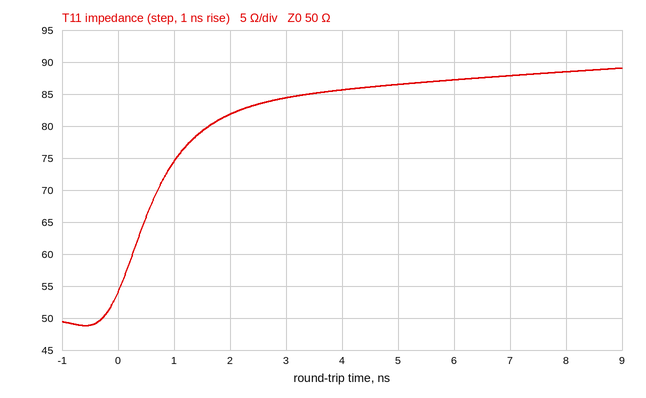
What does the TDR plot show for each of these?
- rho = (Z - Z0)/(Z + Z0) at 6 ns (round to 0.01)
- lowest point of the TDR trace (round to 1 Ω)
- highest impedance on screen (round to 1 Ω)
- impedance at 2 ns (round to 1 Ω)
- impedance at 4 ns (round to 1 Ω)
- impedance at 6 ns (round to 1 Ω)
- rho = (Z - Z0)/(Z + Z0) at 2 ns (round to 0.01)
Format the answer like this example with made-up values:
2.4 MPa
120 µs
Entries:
+0.27
49 Ω
89 Ω
82 Ω
86 Ω
87 Ω
+0.24
